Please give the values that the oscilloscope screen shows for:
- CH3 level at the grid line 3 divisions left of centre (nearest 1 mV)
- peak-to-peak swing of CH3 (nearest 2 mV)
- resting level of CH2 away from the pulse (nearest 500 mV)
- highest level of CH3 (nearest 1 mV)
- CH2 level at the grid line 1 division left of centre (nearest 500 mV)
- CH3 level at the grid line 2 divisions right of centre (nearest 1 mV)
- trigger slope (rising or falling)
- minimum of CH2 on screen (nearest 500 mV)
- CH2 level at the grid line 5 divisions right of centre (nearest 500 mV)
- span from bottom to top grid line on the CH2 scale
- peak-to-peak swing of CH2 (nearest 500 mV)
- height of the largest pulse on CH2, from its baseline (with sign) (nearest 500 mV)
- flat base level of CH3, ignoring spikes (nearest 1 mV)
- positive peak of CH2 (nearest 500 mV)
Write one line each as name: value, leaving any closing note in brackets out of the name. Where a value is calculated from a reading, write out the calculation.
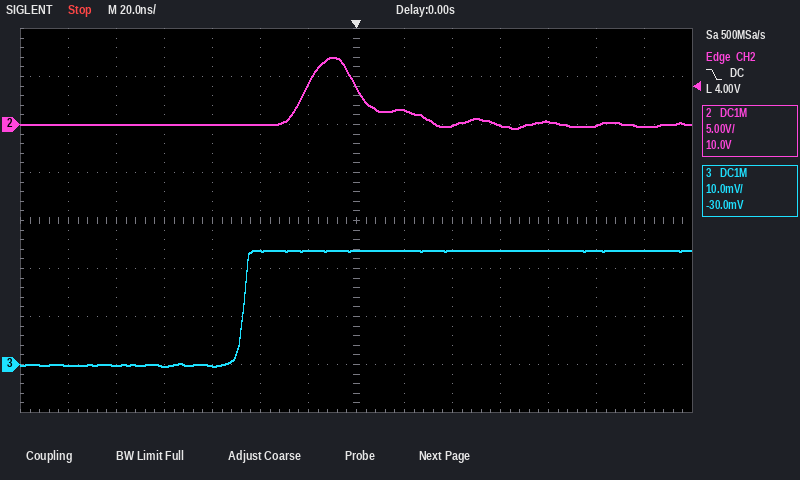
CH3 level at the grid line 3 divisions left of centre: 0 mV
peak-to-peak swing of CH3: 24 mV
resting level of CH2 away from the pulse: 0.0 V
highest level of CH3: 24 mV
CH2 level at the grid line 1 division left of centre: 4.0 V
CH3 level at the grid line 2 divisions right of centre: 24 mV
trigger slope: falling
minimum of CH2 on screen: -500 mV
CH2 level at the grid line 5 divisions right of centre: 0.0 V
span from bottom to top grid line on the CH2 scale: 40 V
peak-to-peak swing of CH2: 7.0 V − (-500 mV) = 7.5 V
height of the largest pulse on CH2, from its baseline (with sign): 7.0 V − (0.0 V) = +7.0 V
flat base level of CH3, ignoring spikes: 0 mV
positive peak of CH2: 7.0 V
